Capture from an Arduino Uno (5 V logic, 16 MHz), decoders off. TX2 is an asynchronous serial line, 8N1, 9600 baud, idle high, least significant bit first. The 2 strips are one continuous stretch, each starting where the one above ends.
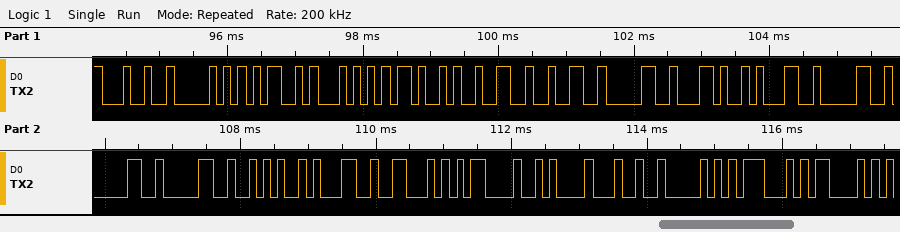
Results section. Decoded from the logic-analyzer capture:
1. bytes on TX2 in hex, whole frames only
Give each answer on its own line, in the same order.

24 50 4D 54 4B 32 32 30 2C 31 30 30 30 2A 31 46 0D 0A 24 50 47 43
